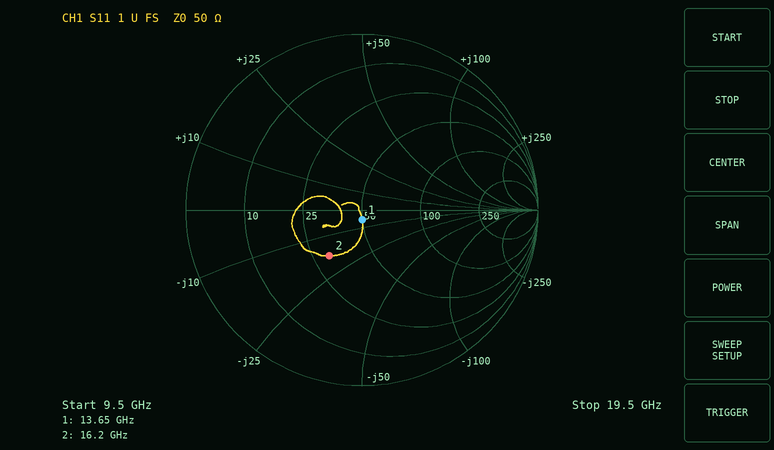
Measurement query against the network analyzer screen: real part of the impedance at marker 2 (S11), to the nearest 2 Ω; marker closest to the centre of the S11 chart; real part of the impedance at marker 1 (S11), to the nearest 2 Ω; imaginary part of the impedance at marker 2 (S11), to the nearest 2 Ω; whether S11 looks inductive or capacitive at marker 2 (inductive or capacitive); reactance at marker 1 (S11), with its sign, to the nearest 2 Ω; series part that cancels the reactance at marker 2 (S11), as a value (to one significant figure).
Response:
30 Ω
marker 1
50 Ω
-18 Ω
capacitive
-6 Ω
200 pH
